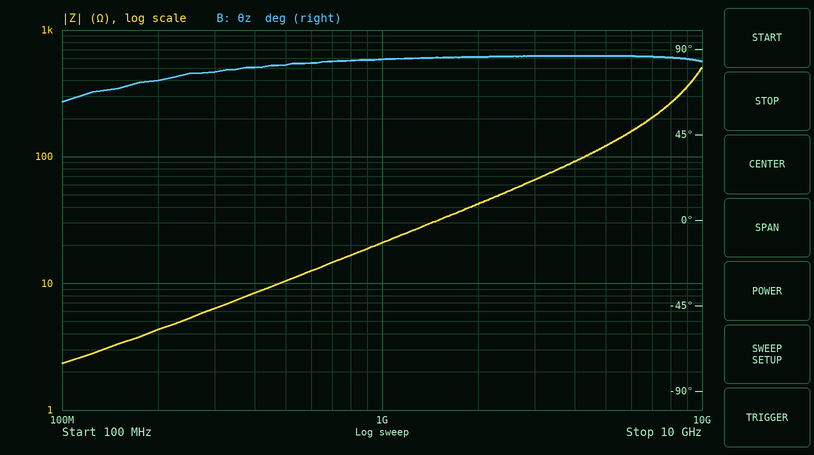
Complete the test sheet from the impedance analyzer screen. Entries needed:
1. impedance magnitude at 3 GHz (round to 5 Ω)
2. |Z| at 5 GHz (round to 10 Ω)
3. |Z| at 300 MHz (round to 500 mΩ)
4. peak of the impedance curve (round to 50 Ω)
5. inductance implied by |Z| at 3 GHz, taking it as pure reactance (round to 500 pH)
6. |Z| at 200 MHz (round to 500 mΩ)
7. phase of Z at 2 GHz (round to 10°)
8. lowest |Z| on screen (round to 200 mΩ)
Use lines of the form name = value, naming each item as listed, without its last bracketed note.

impedance magnitude at 3 GHz = 65 Ω
|Z| at 5 GHz = 120 Ω
|Z| at 300 MHz = 6.5 Ω
peak of the impedance curve = 500 Ω
inductance implied by |Z| at 3 GHz, taking it as pure reactance = 3.5 nH
|Z| at 200 MHz = 4.5 Ω
phase of Z at 2 GHz = 90°
lowest |Z| on screen = 2.4 Ω
